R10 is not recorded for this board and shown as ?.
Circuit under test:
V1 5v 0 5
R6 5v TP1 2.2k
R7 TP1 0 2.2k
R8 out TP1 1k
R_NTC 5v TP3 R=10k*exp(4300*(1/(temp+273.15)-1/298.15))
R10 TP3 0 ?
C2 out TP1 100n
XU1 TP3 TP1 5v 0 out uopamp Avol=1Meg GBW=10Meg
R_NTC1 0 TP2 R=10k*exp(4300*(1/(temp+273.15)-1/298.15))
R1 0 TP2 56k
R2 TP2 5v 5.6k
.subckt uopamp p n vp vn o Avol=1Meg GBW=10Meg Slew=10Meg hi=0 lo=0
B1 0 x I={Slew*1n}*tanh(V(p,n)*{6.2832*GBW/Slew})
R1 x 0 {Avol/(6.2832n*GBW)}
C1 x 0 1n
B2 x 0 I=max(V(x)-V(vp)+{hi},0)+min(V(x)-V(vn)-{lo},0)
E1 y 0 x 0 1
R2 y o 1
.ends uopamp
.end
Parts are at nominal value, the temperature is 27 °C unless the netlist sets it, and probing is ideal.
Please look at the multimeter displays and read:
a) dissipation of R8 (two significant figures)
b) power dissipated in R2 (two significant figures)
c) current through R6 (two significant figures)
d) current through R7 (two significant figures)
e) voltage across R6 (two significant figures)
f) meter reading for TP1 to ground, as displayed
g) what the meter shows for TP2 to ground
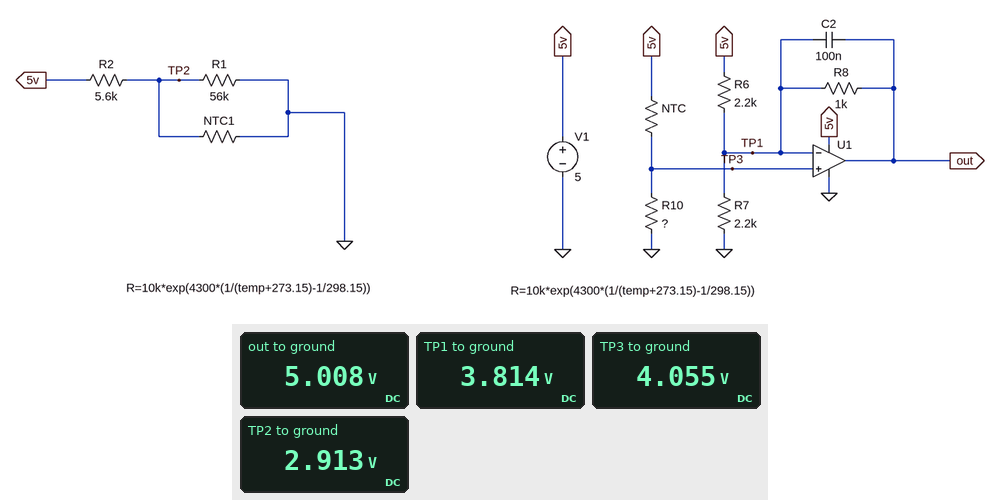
1.4 mW
780 µW
540 µA
1.7 mA
1.2 V
3.814 V
2.913 V
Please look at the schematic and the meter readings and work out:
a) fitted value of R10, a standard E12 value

39 kΩ
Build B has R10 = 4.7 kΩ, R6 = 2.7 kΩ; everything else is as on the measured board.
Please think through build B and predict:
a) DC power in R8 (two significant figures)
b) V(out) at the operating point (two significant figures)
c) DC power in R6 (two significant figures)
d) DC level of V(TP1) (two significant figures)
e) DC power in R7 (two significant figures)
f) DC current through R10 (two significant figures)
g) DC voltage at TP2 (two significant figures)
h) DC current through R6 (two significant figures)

200 µW
1.3 V
4.0 mW
1.7 V
1.3 mW
360 µA
2.9 V
1.2 mA
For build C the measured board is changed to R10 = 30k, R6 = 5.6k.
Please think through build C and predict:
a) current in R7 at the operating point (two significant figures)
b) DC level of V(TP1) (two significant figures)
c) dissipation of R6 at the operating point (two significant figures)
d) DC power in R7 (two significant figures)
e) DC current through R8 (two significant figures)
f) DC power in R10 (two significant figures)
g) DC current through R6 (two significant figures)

1.6 mA
3.6 V
340 µW
5.9 mW
1.4 mA
490 µW
250 µA
